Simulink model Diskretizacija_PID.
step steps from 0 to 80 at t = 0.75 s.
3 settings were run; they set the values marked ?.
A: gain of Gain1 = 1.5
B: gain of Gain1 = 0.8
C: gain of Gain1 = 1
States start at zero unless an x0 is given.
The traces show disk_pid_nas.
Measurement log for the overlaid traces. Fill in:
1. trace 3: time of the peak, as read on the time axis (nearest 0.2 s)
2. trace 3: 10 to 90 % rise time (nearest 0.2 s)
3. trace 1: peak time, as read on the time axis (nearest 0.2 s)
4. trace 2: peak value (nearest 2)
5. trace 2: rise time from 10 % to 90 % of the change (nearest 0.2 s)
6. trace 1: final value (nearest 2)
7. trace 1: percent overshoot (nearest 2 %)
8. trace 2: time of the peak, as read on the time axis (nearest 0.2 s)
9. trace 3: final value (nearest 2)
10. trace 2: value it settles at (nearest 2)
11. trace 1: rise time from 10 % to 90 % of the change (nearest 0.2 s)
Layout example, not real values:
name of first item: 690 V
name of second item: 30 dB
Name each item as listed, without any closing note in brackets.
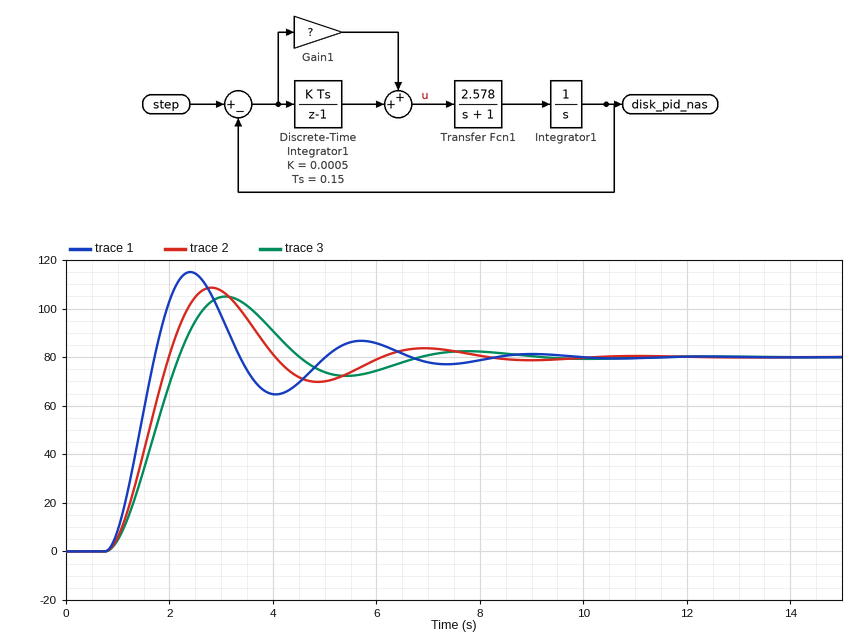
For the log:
trace 3: time of the peak, as read on the time axis: 3.0 s
trace 3: 10 to 90 % rise time: 1.0 s
trace 1: peak time, as read on the time axis: 2.4 s
trace 2: peak value: 108
trace 2: rise time from 10 % to 90 % of the change: 0.8 s
trace 1: final value: 80
trace 1: percent overshoot: 44 %
trace 2: time of the peak, as read on the time axis: 2.8 s
trace 3: final value: 80
trace 2: value it settles at: 80
trace 1: rise time from 10 % to 90 % of the change: 0.6 s
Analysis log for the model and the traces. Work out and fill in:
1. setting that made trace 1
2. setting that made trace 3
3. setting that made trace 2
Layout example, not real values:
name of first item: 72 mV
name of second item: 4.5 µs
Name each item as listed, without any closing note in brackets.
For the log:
setting that made trace 1: A
setting that made trace 3: B
setting that made trace 2: C
